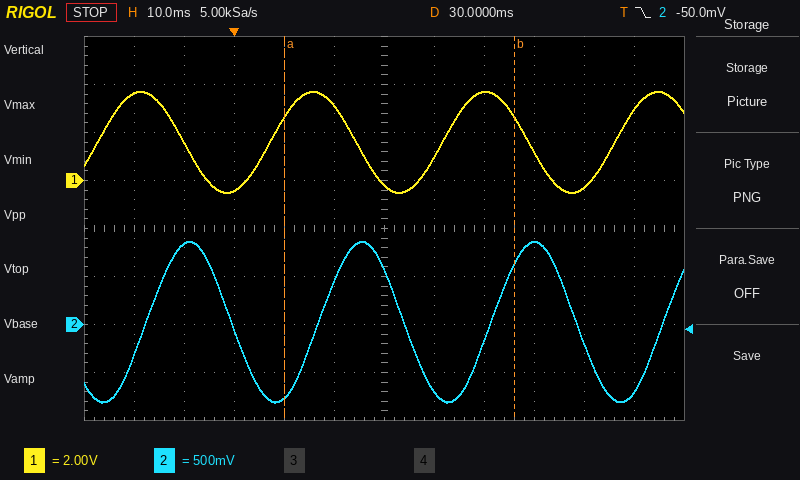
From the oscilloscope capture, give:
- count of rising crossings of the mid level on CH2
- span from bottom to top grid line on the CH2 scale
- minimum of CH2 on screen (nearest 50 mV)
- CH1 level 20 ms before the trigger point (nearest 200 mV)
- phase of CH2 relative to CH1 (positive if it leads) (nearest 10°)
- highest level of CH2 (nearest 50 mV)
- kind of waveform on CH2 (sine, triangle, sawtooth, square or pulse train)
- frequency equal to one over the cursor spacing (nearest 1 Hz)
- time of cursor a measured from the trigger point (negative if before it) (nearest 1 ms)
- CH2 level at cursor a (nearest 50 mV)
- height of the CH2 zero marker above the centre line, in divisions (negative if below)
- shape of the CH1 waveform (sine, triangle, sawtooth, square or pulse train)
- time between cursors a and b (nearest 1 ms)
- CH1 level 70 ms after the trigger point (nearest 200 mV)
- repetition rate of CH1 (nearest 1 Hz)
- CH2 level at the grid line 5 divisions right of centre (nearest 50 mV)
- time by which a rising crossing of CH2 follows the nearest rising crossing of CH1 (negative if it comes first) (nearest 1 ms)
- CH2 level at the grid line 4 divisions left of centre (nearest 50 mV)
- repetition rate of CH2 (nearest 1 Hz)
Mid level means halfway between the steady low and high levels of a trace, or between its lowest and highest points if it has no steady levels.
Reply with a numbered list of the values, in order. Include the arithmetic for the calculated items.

1. 4
2. 4 V
3. -800 mV
4. 3.6 V
5. -100°
6. 850 mV
7. sine
8. 1 / 46 ms ≈ 22 Hz
9. +10 ms
10. -750 mV
11. -2.0 div
12. sine
13. 46 ms
14. -200 mV
15. 29 Hz
16. -700 mV
17. +10 ms
18. 850 mV
19. 29 Hz
